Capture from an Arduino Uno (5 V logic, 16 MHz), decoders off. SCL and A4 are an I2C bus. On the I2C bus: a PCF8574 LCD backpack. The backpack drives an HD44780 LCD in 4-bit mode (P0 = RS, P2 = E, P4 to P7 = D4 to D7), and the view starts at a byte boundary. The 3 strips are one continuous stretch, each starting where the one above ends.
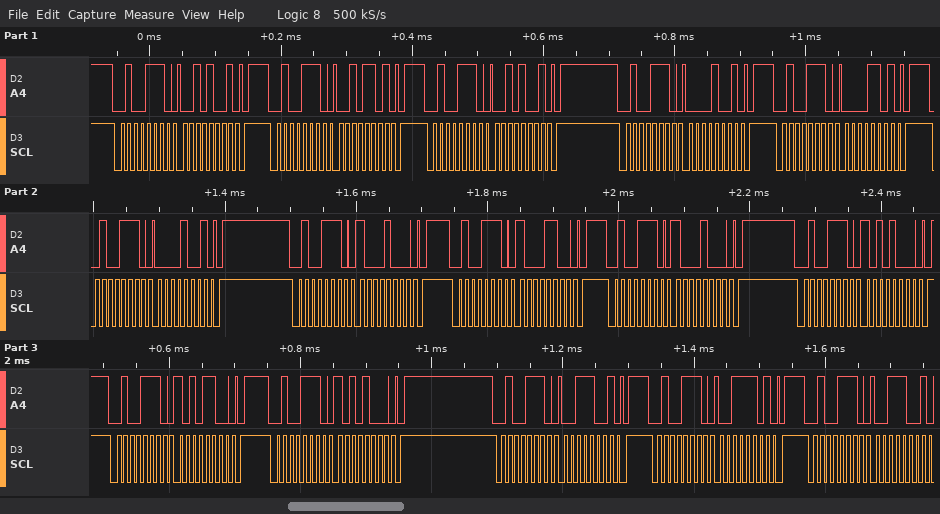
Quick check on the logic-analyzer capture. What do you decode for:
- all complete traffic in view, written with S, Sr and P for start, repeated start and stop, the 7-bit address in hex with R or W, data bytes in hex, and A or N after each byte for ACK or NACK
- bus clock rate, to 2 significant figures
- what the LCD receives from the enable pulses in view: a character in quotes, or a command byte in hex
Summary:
S 27W A 29 A P S 27W A 2D A P S 27W A 29 A P S 27W A 09 A P S 27W A 0D A P S 27W A 09 A P S 27W A 88 A P S 27W A 8C A P S 27W A 88 A P S 27W A A8 A P S 27W A AC A P S 27W A A8 A P S 27W A 39 A P S 27W A 3D A P S 27W A 39 A
100 kHz
' ' 0x8A
